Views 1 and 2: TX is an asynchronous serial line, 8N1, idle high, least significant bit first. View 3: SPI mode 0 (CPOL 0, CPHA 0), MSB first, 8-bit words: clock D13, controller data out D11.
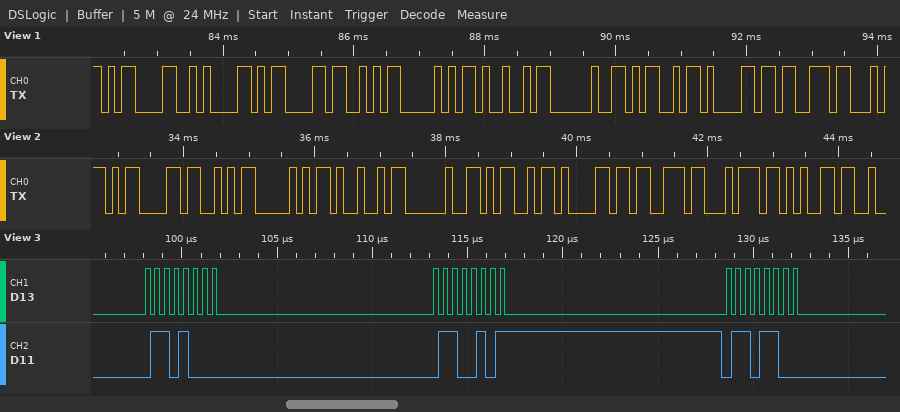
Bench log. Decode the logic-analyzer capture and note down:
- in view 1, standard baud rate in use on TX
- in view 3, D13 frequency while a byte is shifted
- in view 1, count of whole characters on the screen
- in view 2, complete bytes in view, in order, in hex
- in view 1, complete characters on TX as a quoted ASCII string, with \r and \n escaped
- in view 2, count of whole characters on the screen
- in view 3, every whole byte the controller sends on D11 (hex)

9600 baud
2 MHz
10
0D 53 50 49 20 4D 61 73 74 65
"\r\n\rSPI Mas"
10
68 65 6C
